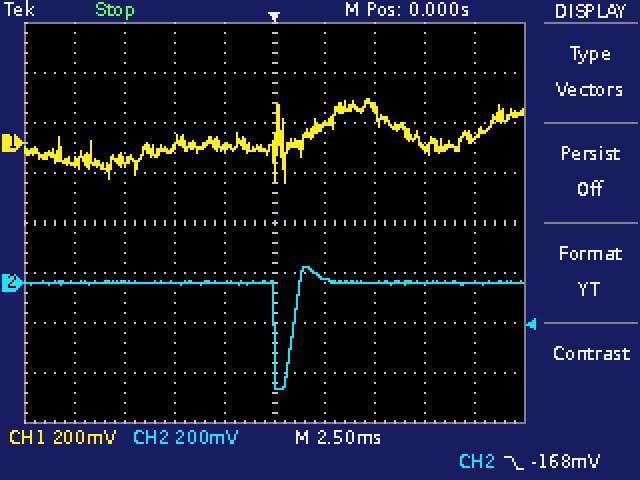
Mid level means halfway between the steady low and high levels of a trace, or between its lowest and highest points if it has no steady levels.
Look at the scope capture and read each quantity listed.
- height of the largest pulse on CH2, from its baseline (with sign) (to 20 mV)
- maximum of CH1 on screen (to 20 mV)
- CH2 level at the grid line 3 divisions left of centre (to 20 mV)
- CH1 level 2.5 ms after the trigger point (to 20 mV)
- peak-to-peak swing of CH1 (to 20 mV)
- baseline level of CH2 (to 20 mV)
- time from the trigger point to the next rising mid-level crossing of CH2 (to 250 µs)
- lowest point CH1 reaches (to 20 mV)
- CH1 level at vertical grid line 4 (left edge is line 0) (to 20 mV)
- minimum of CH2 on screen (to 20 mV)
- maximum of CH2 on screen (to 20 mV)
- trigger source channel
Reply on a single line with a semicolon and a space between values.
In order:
-420 mV; 180 mV; 0 mV; 60 mV; 340 mV; 0 mV; 1.00 ms; -160 mV; -20 mV; -420 mV; 60 mV; CH2
